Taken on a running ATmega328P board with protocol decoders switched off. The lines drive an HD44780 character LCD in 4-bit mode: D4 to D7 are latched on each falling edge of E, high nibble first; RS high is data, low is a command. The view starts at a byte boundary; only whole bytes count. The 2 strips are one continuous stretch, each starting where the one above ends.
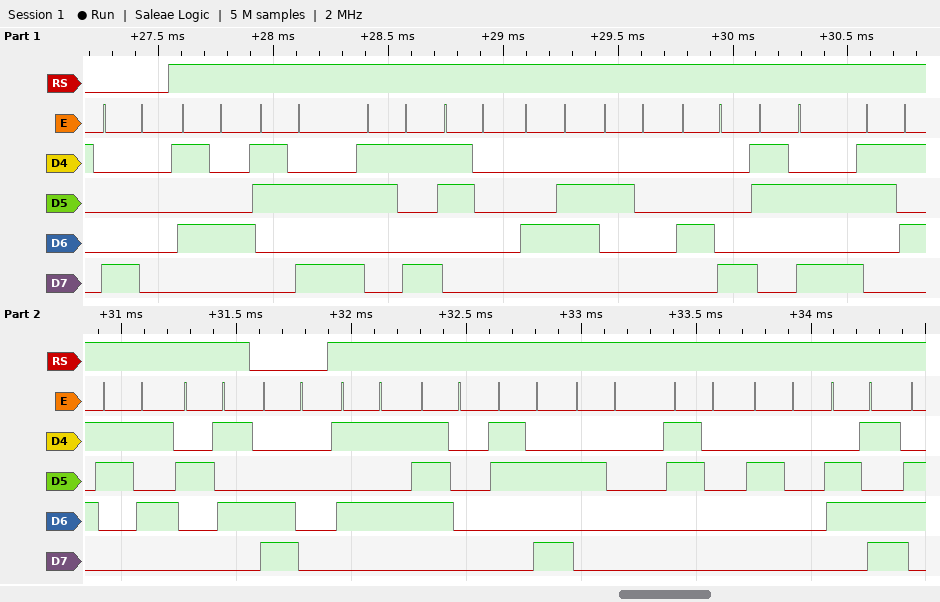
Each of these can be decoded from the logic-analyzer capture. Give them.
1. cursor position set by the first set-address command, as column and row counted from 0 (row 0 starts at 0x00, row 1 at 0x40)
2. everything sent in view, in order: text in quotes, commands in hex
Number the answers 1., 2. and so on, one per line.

1. column 0, row 0
2. 0x80 "T:90F H:55%" 0xC0 "Up: 0 m"
